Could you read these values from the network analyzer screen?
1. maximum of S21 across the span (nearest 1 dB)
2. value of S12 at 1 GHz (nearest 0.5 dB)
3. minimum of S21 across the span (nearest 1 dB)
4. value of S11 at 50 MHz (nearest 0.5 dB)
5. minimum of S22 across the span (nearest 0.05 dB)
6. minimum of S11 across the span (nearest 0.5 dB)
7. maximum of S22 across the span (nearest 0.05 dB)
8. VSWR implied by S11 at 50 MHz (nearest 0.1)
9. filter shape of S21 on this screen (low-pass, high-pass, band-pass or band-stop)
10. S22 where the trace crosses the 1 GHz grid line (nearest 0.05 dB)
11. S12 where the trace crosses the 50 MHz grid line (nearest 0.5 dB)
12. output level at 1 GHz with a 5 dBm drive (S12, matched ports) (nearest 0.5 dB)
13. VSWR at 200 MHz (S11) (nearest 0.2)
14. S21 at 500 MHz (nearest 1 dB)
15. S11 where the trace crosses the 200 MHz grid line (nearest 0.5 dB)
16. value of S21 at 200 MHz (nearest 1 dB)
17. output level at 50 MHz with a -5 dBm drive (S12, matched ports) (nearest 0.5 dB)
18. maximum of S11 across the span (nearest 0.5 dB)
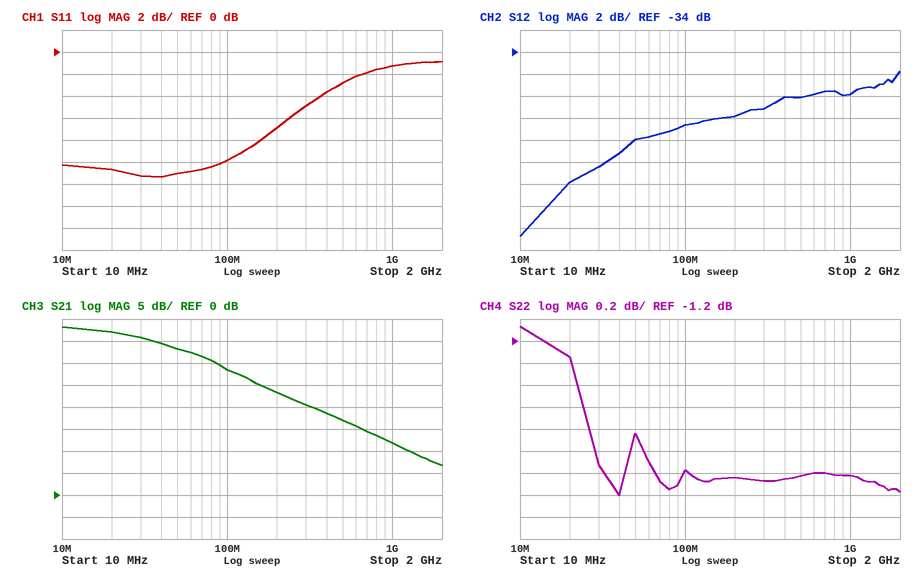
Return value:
38 dB
-38.0 dB
7 dB
-11.0 dB
-2.60 dB
-11.5 dB
-1.05 dB
1.8
low-pass
-2.40 dB
-42.0 dB
-33.0 dBm
2.6
17 dB
-7.0 dB
23 dB
-47.0 dBm
-1.0 dB
